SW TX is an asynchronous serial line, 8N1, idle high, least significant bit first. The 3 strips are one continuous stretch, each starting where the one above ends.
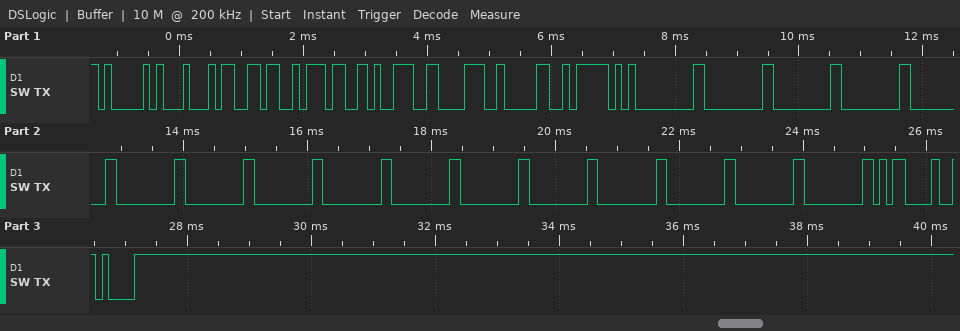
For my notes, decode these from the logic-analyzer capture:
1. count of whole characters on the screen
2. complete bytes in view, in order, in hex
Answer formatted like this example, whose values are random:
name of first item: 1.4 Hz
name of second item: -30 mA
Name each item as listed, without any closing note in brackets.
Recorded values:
count of whole characters on the screen: 26
complete bytes in view, in order, in hex: 41 44 36 37 39 38 30 5F 00 00 00 00 00 00 00 00 00 00 00 00 00 00 00 00 0D 0A
